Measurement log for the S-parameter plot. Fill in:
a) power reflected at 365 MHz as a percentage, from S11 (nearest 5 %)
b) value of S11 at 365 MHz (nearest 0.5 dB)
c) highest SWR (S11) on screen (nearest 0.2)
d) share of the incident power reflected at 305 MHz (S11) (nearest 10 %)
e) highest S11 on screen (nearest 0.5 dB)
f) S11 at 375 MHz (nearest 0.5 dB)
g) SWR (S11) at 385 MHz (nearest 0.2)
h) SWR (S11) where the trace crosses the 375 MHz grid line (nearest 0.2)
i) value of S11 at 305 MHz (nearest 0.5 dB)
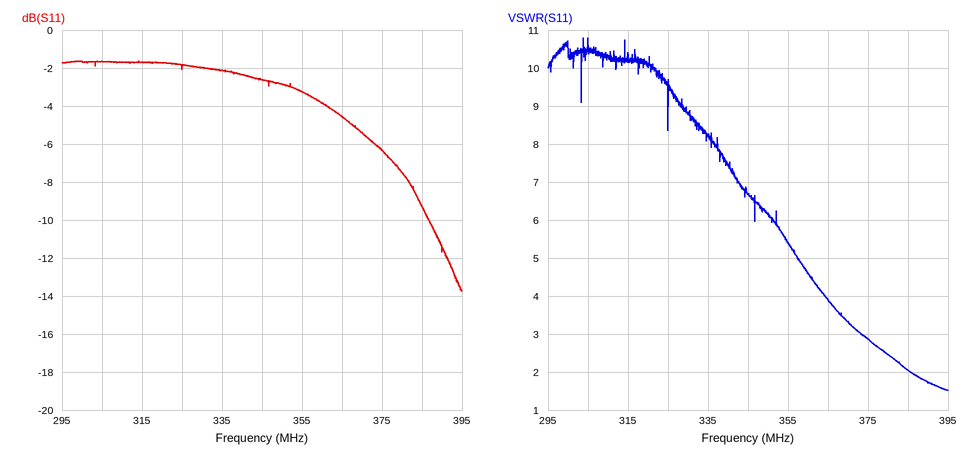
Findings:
35 %
-4.5 dB
10.8
70 %
-1.5 dB
-6.5 dB
2.0
2.8
-1.5 dB
